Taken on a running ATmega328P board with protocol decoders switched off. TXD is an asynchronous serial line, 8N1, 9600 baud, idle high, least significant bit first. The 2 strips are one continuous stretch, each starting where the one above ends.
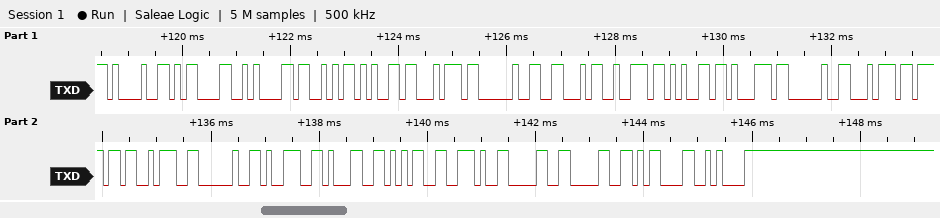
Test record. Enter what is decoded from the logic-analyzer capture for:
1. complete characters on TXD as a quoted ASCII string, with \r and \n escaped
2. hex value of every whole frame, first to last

"!\r\nSet Freq to: 915.00\r\n"
21 0D 0A 53 65 74 20 46 72 65 71 20 74 6F 3A 20 39 31 35 2E 30 30 0D 0A
